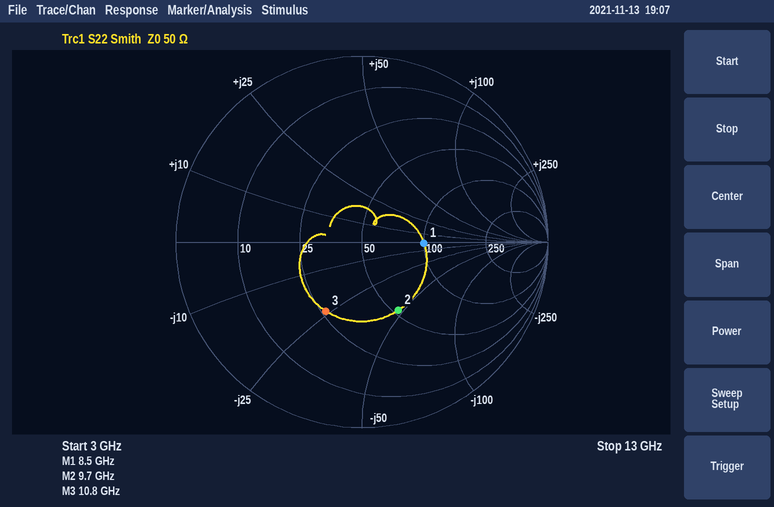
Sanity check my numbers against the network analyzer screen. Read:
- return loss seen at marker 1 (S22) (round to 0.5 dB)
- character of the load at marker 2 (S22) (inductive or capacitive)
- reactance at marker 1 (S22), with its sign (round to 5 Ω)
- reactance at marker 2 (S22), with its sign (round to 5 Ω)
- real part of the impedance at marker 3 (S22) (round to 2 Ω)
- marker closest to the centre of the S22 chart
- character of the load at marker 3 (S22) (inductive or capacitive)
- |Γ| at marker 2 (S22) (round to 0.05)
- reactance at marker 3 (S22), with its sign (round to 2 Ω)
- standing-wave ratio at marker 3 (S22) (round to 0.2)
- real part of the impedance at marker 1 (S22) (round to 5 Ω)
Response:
9.5 dB
capacitive
0 Ω
-45 Ω
26 Ω
marker 1
capacitive
0.40
-24 Ω
2.4
100 Ω
